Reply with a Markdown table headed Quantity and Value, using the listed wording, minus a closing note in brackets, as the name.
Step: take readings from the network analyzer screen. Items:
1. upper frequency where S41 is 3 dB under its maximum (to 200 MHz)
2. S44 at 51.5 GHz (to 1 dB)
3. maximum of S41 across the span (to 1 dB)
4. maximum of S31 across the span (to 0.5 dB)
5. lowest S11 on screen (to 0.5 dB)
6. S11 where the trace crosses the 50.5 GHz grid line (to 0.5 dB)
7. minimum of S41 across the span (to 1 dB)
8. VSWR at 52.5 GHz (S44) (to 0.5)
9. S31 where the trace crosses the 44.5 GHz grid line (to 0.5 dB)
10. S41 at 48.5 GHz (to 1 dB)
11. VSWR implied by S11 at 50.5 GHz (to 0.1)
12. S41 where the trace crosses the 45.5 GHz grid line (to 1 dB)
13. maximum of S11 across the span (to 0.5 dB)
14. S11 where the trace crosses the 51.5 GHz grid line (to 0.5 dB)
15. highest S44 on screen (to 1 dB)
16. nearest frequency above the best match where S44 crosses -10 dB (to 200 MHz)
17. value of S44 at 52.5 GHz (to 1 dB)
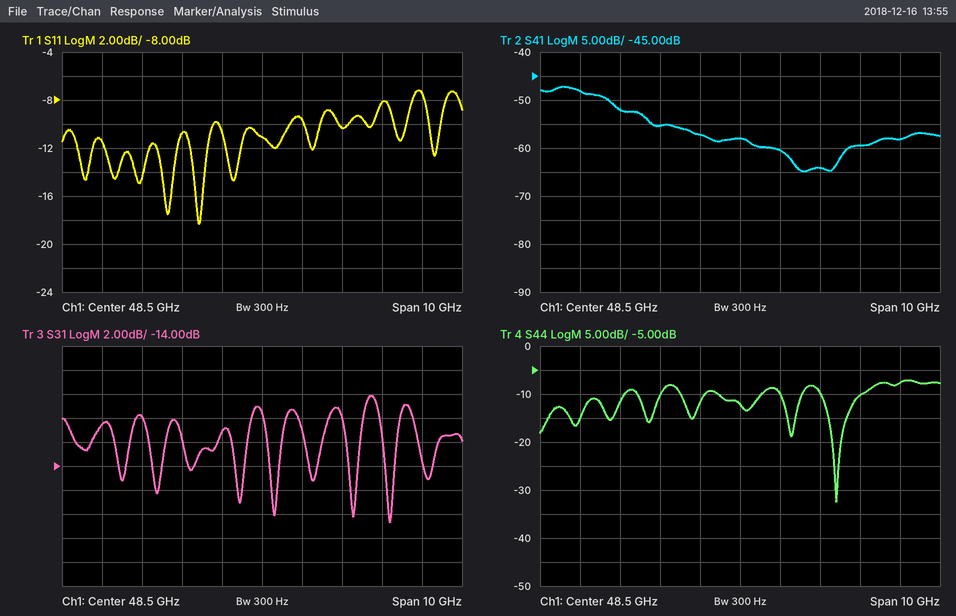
| Quantity | Value |
|---|---|
| upper frequency where S41 is 3 dB under its maximum | 45.2 GHz |
| S44 at 51.5 GHz | -10 dB |
| maximum of S41 across the span | -47 dB |
| maximum of S31 across the span | -8.0 dB |
| lowest S11 on screen | -18.5 dB |
| S11 where the trace crosses the 50.5 GHz grid line | -10.5 dB |
| minimum of S41 across the span | -65 dB |
| VSWR at 52.5 GHz (S44) | 2.5 |
| S31 where the trace crosses the 44.5 GHz grid line | -10.5 dB |
| S41 at 48.5 GHz | -58 dB |
| VSWR implied by S11 at 50.5 GHz | 1.9 |
| S41 where the trace crosses the 45.5 GHz grid line | -52 dB |
| maximum of S11 across the span | -7.0 dB |
| S11 where the trace crosses the 51.5 GHz grid line | -8.0 dB |
| highest S44 on screen | -7 dB |
| nearest frequency above the best match where S44 crosses -10 dB | 51.6 GHz |
| value of S44 at 52.5 GHz | -8 dB |
